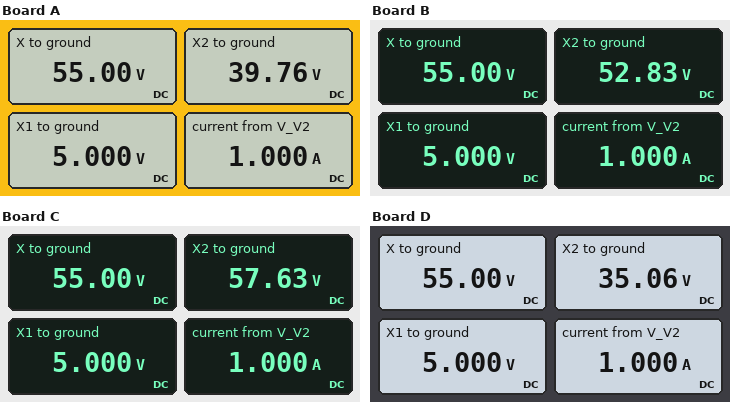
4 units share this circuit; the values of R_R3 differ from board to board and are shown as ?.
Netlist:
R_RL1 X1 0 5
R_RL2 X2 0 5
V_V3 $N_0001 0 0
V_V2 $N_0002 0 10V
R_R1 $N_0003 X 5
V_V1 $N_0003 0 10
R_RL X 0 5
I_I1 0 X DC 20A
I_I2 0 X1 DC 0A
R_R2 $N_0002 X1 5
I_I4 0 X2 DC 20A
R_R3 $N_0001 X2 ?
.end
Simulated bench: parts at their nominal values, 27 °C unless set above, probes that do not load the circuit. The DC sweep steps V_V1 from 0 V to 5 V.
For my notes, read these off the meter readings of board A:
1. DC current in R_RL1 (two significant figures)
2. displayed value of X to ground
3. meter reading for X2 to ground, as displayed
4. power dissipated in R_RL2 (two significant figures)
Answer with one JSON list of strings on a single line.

["1.0 A", "55.00 V", "39.76 V", "320 W"]
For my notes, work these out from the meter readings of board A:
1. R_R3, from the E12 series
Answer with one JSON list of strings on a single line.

["3.3 Ω"]
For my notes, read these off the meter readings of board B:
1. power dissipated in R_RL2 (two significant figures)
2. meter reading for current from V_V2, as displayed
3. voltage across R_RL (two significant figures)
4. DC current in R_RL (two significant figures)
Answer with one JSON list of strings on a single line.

["560 W", "1.000 A", "55 V", "11 A"]
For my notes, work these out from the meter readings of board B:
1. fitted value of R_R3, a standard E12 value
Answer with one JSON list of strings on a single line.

["5.6 Ω"]
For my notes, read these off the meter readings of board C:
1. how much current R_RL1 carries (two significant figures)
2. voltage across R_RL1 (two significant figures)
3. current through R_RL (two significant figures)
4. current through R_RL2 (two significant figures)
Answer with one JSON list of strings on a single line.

["1.0 A", "5.0 V", "11 A", "12 A"]
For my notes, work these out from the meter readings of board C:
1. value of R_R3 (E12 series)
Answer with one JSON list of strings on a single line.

["6.8 Ω"]
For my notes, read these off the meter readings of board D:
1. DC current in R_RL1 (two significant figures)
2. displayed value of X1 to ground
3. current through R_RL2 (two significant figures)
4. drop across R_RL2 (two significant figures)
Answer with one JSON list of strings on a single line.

["1.0 A", "5.000 V", "7.0 A", "35 V"]
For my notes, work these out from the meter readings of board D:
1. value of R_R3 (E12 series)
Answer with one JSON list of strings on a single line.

["2.7 Ω"]
